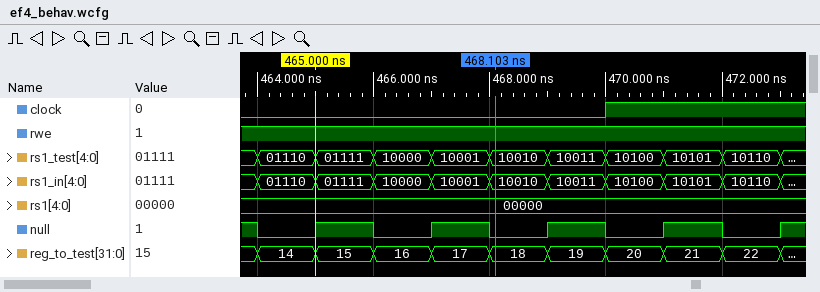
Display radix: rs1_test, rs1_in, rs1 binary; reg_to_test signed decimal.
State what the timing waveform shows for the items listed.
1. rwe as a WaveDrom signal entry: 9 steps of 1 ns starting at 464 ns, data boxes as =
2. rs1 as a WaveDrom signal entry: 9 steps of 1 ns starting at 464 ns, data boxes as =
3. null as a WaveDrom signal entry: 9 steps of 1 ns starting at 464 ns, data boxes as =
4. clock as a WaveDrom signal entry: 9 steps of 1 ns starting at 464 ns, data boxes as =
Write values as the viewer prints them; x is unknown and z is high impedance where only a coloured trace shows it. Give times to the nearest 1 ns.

{name: 'rwe', wave: '1........'}
{name: 'rs1', wave: '=........', data: '00000'}
{name: 'null', wave: '010101010'}
{name: 'clock', wave: '0.....1..'}
